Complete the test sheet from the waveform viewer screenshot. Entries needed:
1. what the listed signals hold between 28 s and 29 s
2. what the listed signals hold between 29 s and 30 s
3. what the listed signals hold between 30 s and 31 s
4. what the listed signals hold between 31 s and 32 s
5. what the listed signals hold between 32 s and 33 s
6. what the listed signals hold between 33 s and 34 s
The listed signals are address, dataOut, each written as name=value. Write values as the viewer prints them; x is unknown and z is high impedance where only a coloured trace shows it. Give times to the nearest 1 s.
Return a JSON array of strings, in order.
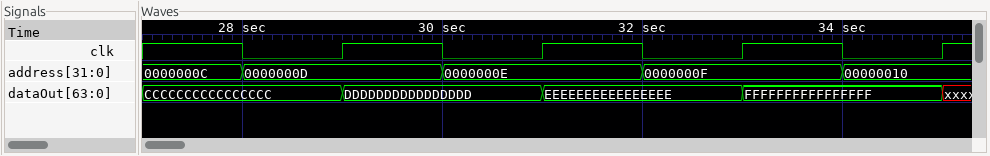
["address=0000000D, dataOut=CCCCCCCCCCCCCCCC", "address=0000000D, dataOut=DDDDDDDDDDDDDDDD", "address=0000000E, dataOut=DDDDDDDDDDDDDDDD", "address=0000000E, dataOut=EEEEEEEEEEEEEEEE", "address=0000000F, dataOut=EEEEEEEEEEEEEEEE", "address=0000000F, dataOut=FFFFFFFFFFFFFFFF"]
